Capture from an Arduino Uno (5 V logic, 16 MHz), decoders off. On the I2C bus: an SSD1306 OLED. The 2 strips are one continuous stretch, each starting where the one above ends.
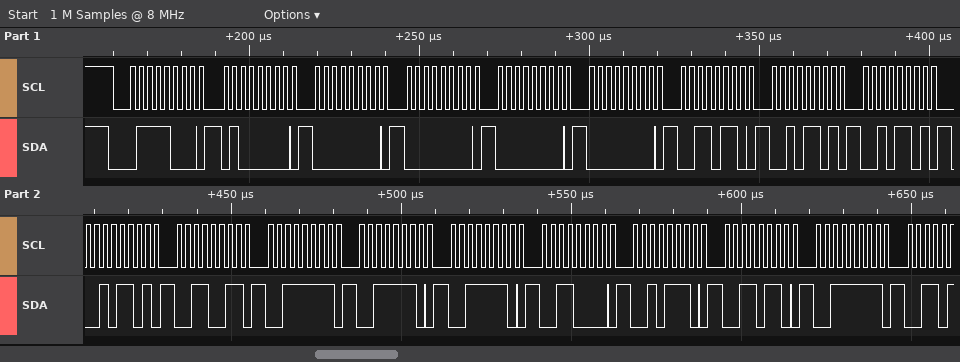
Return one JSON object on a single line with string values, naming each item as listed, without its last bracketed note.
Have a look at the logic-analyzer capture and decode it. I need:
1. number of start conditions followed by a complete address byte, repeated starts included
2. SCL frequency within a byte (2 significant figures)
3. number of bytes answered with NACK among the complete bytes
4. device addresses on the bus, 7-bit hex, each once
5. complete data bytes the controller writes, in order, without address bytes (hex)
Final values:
{"number of start conditions followed by a complete address byte, repeated starts included": "1", "SCL frequency within a byte": "400 kHz", "number of bytes answered with NACK among the complete bytes": "0", "device addresses on the bus, 7-bit hex, each once": "0x3C", "complete data bytes the controller writes, in order, without address bytes": "40 00 00 00 00 36 2D 2D 2D 33 3F 3E 3E 30 2E 36 3F"}
